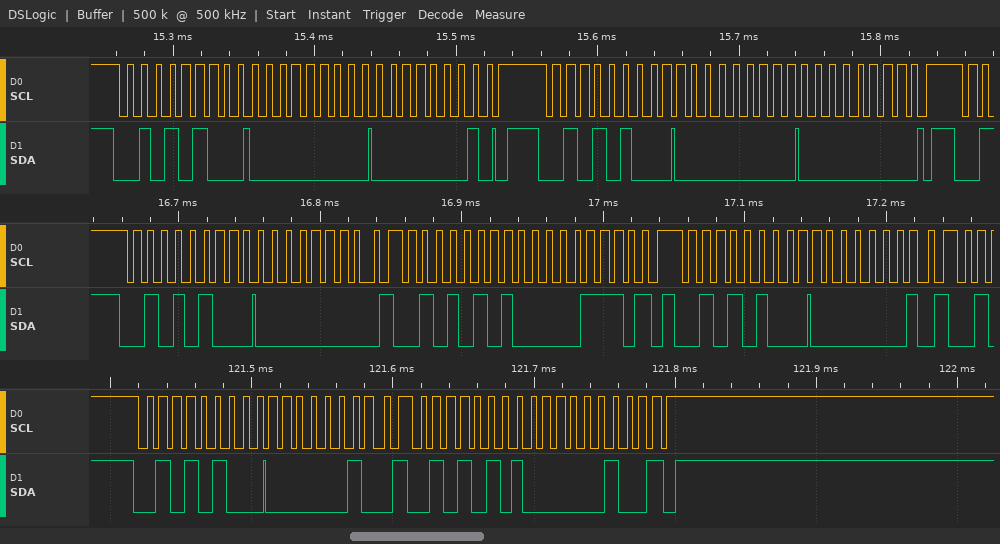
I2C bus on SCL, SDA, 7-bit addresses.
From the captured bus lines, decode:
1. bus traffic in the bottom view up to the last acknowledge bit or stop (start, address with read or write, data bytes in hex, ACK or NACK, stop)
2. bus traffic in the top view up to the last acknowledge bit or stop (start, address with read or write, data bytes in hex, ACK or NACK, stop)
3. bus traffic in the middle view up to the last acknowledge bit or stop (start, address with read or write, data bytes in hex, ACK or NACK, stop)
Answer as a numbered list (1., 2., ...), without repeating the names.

1. start, address 2A write ACK, 02 ACK, repeated start, address 2A read ACK, 04 NACK, stop
2. start, address 2A write ACK, 00 ACK, 01 ACK, stop, start, address 2A write ACK, 00 ACK, 00 ACK, stop
3. start, address 2A write ACK, 00 ACK, repeated start, address 2A read ACK, 0E NACK, stop, start, address 2A write ACK, 01 ACK
